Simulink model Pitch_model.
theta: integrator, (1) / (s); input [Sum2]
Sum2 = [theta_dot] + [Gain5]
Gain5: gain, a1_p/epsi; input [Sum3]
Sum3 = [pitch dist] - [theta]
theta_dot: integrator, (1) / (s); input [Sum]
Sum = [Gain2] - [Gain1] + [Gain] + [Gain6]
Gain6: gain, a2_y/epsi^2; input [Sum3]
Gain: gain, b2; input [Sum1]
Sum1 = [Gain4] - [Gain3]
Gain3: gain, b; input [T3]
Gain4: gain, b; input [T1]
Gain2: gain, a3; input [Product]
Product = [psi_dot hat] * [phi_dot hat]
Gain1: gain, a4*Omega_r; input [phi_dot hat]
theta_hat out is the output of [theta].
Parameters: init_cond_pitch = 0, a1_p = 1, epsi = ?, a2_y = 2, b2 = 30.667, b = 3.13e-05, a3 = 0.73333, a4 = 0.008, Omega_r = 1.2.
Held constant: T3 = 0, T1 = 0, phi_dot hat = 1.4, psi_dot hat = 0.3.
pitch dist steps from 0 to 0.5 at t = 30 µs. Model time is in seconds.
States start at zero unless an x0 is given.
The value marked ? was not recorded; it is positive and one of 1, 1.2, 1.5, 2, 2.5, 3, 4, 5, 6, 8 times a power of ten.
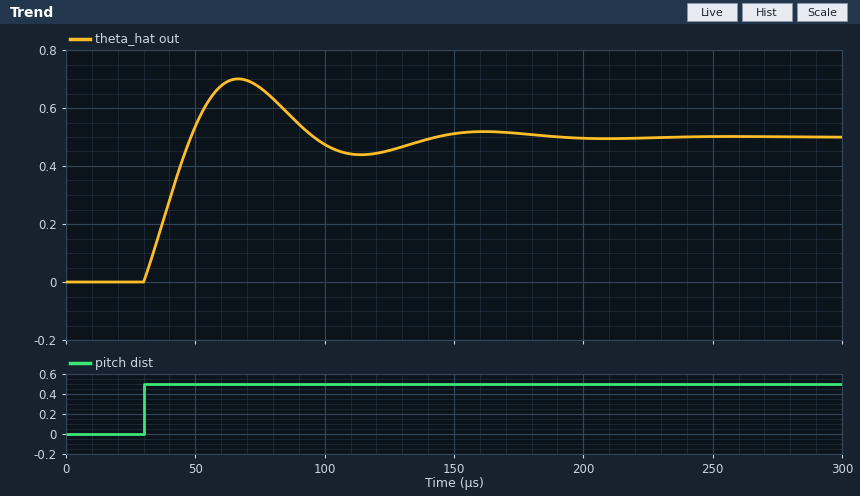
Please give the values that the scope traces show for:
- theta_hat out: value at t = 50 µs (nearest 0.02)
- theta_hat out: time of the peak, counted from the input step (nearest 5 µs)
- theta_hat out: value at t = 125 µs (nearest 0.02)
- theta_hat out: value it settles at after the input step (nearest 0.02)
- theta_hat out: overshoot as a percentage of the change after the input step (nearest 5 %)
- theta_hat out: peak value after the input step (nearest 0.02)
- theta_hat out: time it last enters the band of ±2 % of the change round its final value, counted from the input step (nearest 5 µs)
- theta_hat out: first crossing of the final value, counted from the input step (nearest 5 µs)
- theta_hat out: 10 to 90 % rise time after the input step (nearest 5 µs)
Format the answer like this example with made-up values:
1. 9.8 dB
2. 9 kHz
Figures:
1. 0.54
2. 35 µs
3. 0.46
4. 0.50
5. 40 %
6. 0.70
7. 150 µs
8. 20 µs
9. 15 µs
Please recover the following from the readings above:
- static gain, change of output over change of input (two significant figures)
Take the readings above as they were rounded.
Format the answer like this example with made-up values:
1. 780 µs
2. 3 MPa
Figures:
1. 1.0
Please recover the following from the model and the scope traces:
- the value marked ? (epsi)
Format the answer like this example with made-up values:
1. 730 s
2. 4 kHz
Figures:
1. 2e-05
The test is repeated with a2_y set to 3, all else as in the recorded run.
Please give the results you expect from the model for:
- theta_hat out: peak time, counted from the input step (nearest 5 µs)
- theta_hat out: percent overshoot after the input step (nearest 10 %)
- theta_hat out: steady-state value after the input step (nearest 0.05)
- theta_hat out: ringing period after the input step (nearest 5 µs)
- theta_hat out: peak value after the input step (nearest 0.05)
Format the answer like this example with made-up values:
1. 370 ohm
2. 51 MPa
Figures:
1. 30 µs
2. 50 %
3. 0.50
4. 75 µs
5. 0.75
